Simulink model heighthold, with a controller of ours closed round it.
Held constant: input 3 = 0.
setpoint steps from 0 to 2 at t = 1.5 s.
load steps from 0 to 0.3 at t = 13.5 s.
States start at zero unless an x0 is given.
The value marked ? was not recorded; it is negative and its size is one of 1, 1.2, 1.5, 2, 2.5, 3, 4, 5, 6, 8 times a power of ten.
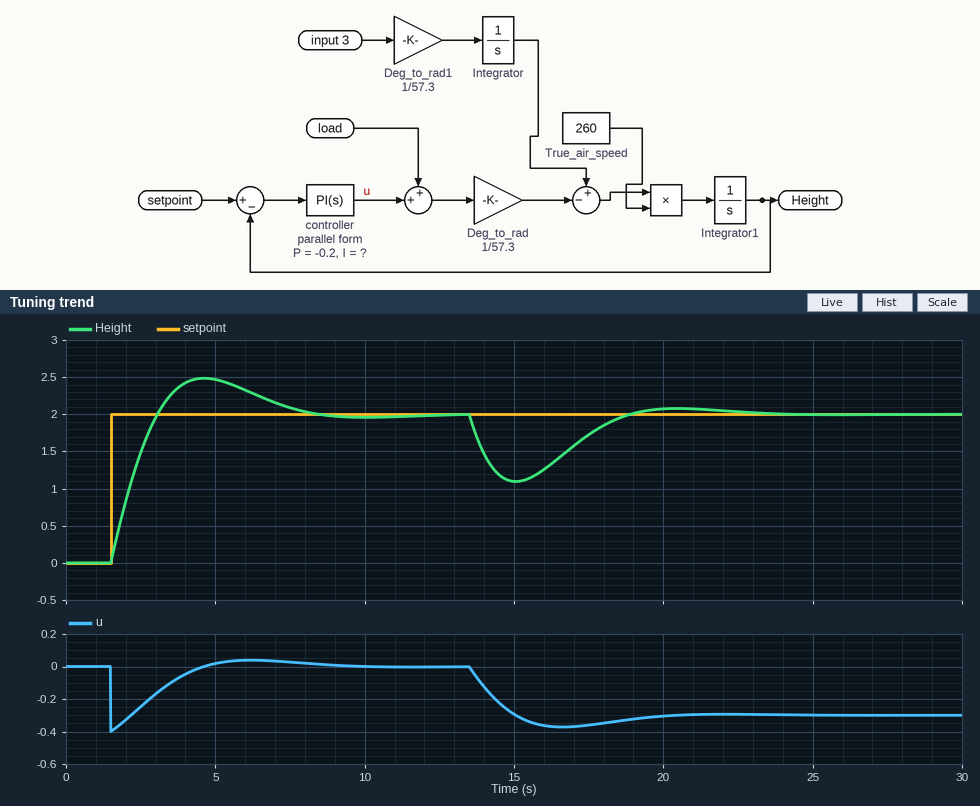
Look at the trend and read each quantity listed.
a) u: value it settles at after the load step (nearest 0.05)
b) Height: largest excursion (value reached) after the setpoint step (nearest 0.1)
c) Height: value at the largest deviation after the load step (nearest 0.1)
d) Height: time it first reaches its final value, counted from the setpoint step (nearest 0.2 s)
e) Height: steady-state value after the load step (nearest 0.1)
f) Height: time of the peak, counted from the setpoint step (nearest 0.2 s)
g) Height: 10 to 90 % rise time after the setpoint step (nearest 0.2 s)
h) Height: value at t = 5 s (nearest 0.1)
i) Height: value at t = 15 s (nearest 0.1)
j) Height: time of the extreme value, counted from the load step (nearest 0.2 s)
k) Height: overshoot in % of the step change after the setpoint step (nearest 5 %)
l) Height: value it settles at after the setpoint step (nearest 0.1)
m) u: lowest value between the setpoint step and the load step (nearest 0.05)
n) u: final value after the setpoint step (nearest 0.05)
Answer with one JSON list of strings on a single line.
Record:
["-0.30", "2.5", "1.1", "1.6 s", "2.0", "3.2 s", "1.2 s", "2.5", "1.1", "1.6 s", "25 %", "2.0", "-0.40", "0.00"]
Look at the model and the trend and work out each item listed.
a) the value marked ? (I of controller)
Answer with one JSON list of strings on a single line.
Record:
["-0.12"]
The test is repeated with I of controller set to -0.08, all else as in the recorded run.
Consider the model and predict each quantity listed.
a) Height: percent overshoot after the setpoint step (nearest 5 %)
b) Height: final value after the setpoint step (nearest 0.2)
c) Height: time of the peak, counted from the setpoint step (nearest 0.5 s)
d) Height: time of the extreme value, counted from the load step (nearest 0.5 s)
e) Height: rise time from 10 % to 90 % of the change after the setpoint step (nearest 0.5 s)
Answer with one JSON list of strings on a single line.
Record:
["20 %", "2.0", "3.5 s", "2.0 s", "1.5 s"]
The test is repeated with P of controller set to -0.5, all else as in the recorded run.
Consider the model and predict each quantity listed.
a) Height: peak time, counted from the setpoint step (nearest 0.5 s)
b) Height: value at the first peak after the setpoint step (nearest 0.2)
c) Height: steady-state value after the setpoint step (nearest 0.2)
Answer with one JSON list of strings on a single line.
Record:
["2.5 s", "2.2", "2.0"]
